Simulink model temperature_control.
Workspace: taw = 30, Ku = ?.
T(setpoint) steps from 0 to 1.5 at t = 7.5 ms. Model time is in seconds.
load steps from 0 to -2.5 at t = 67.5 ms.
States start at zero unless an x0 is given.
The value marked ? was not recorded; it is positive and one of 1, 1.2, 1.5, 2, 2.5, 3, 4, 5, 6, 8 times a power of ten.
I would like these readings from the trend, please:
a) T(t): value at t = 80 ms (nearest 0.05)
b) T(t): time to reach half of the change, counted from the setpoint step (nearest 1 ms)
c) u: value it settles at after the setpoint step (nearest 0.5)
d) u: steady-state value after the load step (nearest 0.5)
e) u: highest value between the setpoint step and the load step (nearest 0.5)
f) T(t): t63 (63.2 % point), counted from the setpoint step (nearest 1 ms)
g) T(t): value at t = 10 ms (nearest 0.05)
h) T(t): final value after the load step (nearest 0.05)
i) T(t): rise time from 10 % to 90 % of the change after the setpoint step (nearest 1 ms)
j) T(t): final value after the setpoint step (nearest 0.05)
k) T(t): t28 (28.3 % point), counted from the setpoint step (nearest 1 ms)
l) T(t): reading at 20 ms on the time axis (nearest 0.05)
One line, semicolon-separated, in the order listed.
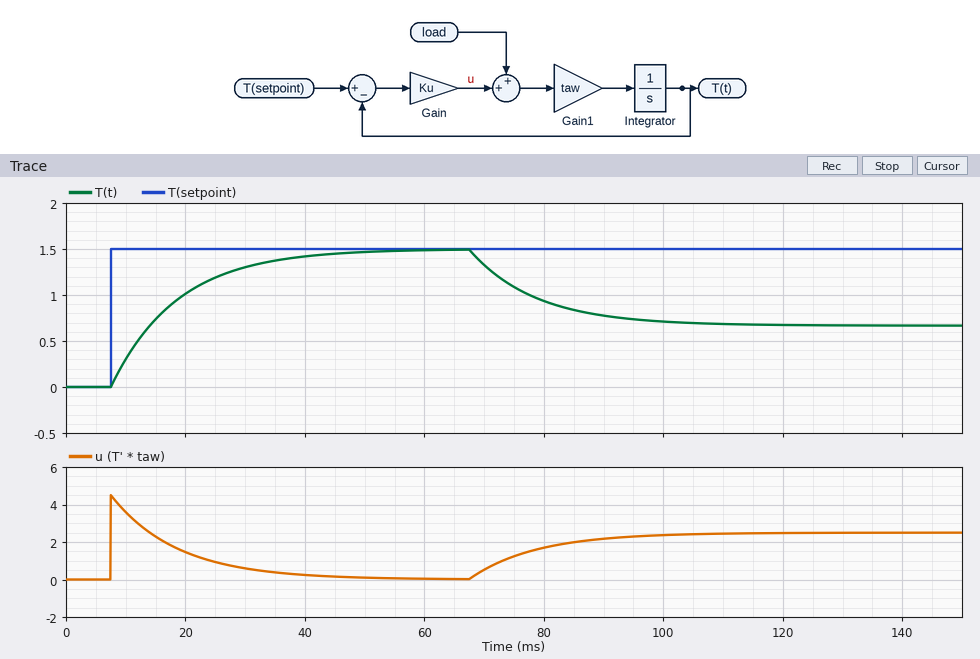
0.95; 8 ms; 0.0; 2.5; 4.5; 11 ms; 0.30; 0.65; 24 ms; 1.50; 4 ms; 1.00
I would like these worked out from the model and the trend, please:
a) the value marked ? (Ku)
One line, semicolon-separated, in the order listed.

3
